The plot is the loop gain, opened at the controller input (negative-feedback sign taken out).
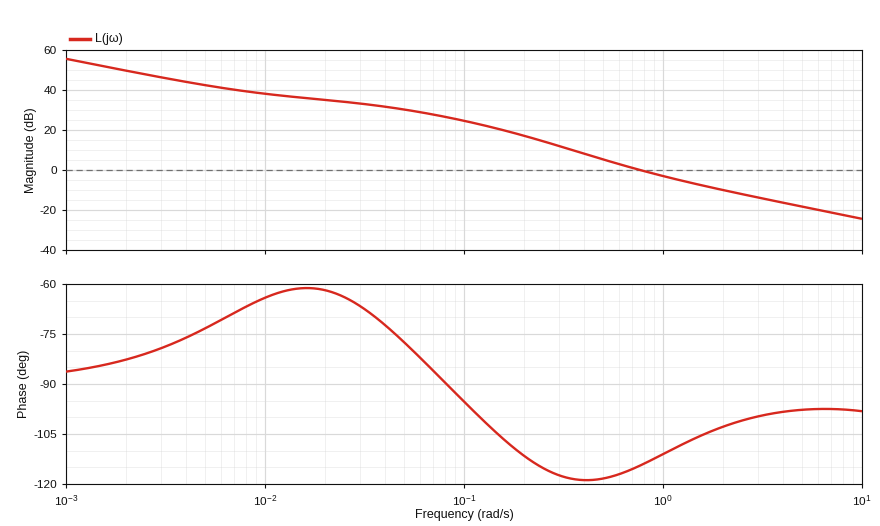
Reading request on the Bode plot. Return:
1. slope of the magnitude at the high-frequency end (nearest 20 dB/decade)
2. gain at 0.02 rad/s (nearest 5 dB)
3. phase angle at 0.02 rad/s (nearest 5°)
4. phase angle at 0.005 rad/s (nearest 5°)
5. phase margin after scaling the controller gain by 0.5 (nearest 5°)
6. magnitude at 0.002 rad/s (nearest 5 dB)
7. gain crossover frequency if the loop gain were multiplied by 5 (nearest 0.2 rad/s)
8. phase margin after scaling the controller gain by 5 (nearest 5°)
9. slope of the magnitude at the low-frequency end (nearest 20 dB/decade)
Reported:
-20 dB/decade
35 dB
-60°
-75°
60°
50 dB
3.0 rad/s
80°
-20 dB/decade
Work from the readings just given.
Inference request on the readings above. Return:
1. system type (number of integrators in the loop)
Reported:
1
